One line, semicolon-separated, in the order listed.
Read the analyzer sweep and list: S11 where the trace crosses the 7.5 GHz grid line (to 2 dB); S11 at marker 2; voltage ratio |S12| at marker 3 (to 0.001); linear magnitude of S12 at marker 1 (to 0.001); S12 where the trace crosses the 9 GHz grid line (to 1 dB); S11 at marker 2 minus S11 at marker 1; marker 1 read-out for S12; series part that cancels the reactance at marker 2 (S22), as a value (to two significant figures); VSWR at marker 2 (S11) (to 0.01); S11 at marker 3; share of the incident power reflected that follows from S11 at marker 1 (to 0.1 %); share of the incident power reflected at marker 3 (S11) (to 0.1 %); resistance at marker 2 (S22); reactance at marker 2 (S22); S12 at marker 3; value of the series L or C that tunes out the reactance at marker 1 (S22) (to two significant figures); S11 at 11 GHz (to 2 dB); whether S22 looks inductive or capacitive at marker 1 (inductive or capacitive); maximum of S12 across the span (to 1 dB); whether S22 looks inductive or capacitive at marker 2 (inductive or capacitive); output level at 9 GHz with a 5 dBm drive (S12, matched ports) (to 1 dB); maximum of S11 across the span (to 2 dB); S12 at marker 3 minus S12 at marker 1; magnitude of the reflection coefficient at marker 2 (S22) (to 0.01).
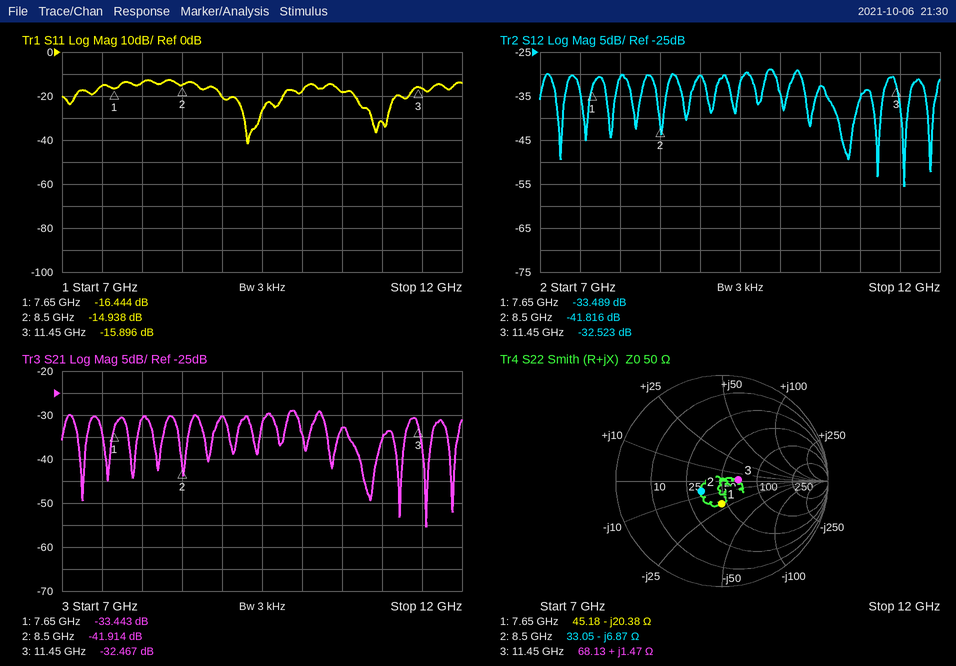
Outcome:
-16 dB; -14.938 dB; 0.024; 0.021; -30 dB; 1.506 dB; -33.489 dB; 130 pH; 1.44; -15.896 dB; 2.3 %; 2.6 %; 33.05 Ω; -6.87 Ω; -32.523 dB; 420 pH; -32 dB; capacitive; -29 dB; capacitive; -25 dBm; -12 dB; 0.966 dB; 0.22
